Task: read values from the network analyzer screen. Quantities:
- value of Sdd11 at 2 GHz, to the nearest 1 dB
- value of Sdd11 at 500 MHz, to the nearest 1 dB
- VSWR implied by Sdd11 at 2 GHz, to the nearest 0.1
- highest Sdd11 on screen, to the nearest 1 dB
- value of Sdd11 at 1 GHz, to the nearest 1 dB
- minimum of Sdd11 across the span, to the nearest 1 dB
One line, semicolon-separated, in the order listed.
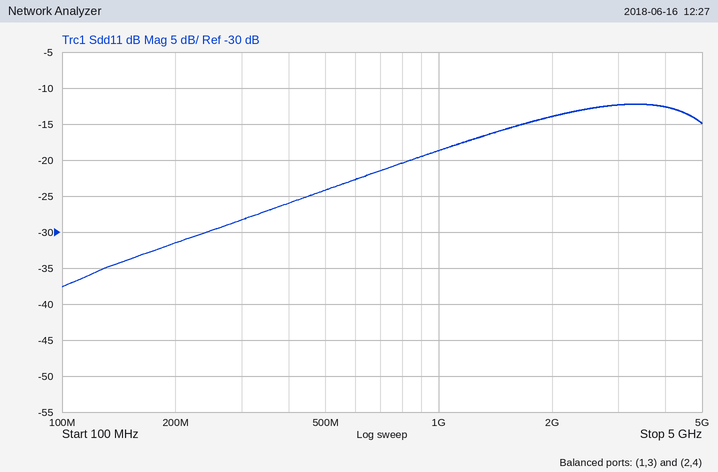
-14 dB; -24 dB; 1.5; -12 dB; -19 dB; -38 dB
